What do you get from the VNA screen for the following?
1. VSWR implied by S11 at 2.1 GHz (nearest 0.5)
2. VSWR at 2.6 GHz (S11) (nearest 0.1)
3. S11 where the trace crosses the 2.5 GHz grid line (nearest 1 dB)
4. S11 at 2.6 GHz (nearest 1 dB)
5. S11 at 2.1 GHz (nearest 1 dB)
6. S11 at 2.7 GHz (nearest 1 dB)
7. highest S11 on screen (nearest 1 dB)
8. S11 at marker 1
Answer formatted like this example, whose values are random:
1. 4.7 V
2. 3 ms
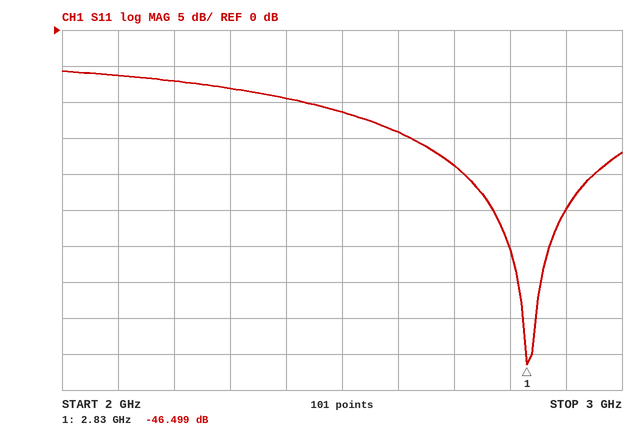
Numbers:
1. 3.0
2. 1.5
3. -11 dB
4. -14 dB
5. -6 dB
6. -19 dB
7. -6 dB
8. -46.499 dB
